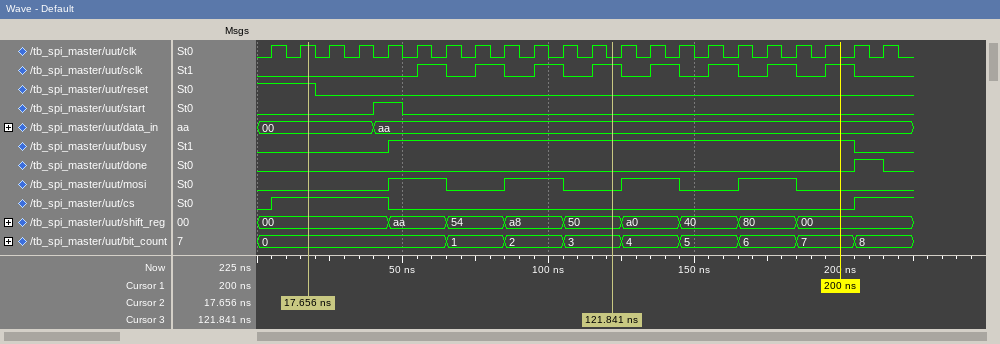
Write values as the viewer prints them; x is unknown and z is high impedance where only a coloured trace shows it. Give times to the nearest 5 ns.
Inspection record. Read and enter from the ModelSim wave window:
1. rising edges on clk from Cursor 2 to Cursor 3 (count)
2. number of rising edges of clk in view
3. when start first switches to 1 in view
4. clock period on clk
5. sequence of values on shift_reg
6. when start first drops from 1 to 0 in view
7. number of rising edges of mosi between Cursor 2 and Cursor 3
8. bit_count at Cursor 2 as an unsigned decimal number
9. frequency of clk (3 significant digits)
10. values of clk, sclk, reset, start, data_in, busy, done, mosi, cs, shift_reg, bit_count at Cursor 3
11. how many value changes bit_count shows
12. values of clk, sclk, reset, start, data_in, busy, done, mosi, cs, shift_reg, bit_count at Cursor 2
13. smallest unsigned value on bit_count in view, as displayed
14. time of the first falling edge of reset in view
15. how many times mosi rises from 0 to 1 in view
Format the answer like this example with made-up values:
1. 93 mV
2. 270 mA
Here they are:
1. 10
2. 22
3. 40 ns
4. 10 ns
5. 00, aa, 54, a8, 50, a0, 40, 80, 00
6. 50 ns
7. 2
8. 0
9. 100 MHz
10. clk=0, sclk=1, reset=0, start=0, data_in=aa, busy=1, done=0, mosi=0, cs=0, shift_reg=50, bit_count=3
11. 8
12. clk=1, sclk=0, reset=1, start=0, data_in=00, busy=0, done=0, mosi=0, cs=1, shift_reg=00, bit_count=0
13. 0
14. 20 ns
15. 4
